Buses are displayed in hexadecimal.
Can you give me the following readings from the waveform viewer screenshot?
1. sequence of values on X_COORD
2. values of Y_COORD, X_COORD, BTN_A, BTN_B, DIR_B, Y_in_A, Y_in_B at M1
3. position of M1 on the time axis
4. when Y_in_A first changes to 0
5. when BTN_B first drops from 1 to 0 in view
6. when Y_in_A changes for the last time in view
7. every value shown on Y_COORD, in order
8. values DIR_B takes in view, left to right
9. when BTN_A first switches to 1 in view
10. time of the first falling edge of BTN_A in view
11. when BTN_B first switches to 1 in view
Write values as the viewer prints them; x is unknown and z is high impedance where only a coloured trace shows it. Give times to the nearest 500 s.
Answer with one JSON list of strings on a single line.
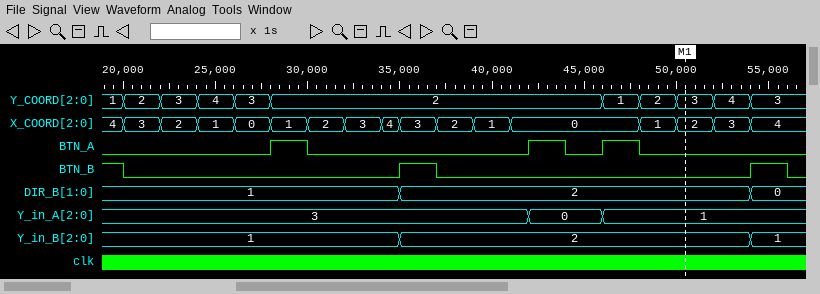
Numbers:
["4, 3, 2, 1, 0, 1, 2, 3, 4, 3, 2, 1, 0, 1, 2, 3, 4", "Y_COORD=3, X_COORD=2, BTN_A=0, BTN_B=0, DIR_B=2, Y_in_A=1, Y_in_B=2", "50500 s", "42000 s", "20000 s", "46000 s", "1, 2, 3, 4, 3, 2, 1, 2, 3, 4, 3", "1, 2, 0", "28000 s", "30000 s", "35000 s"]
